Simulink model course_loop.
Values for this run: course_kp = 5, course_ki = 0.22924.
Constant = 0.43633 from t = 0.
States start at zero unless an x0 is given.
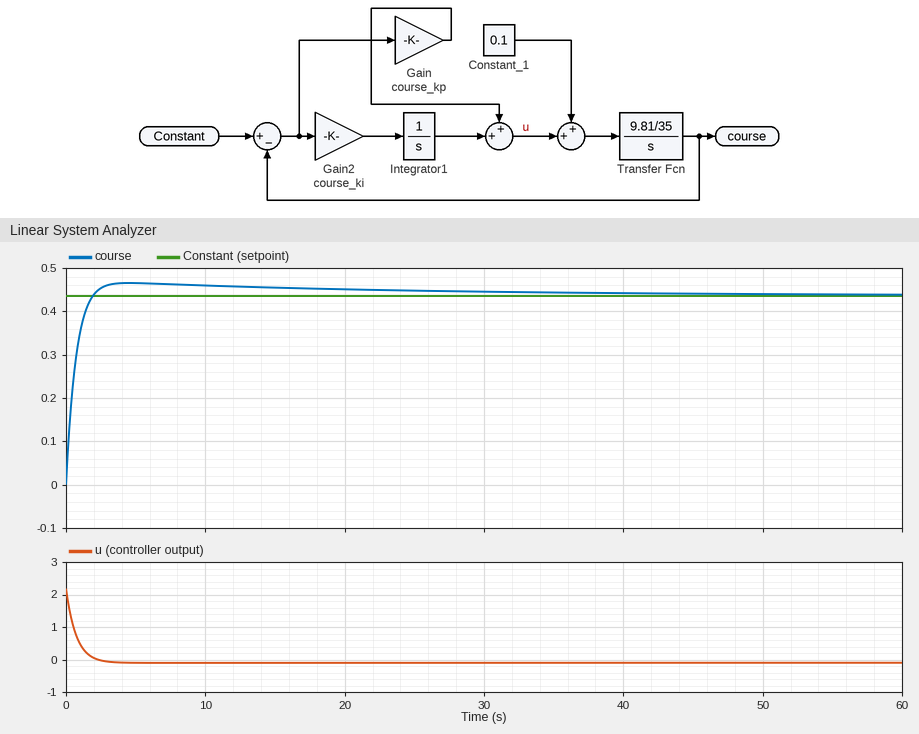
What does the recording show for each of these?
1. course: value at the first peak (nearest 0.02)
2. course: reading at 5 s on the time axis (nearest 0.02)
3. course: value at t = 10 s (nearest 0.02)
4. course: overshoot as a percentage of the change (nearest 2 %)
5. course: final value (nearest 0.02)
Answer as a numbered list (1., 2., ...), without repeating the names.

1. 0.46
2. 0.46
3. 0.46
4. 6 %
5. 0.44
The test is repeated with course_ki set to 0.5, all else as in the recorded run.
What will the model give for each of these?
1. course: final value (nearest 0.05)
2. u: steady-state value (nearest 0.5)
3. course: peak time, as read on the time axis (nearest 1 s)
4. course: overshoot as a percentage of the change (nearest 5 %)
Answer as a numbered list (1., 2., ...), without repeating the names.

1. 0.45
2. 0.0
3. 4 s
4. 10 %
